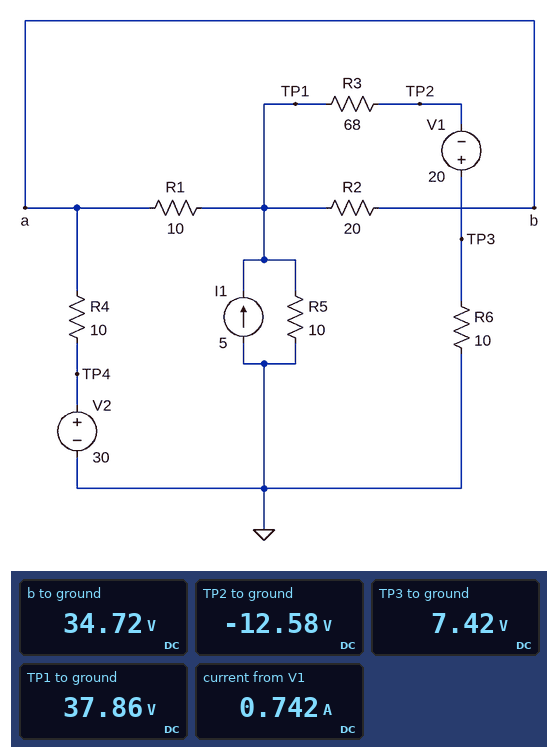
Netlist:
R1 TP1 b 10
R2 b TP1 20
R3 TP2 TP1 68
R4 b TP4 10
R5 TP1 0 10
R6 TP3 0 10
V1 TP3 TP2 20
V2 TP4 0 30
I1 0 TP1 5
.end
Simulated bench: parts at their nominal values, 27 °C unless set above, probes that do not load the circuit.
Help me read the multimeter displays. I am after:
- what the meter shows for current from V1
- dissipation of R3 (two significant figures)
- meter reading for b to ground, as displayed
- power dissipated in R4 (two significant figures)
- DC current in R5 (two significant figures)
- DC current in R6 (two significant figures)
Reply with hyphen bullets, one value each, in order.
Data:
- 0.742 A
- 37 W
- 34.72 V
- 2.2 W
- 3.8 A
- 740 mA
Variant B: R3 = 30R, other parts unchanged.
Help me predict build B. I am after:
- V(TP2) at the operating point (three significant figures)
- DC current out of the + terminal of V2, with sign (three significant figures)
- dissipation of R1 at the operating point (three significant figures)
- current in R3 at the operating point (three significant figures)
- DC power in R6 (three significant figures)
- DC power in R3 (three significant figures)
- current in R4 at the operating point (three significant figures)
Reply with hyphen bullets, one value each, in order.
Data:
- -6.49 V
- -243 mA
- 263 mW
- 1.35 A
- 18.3 W
- 54.8 W
- 243 mA
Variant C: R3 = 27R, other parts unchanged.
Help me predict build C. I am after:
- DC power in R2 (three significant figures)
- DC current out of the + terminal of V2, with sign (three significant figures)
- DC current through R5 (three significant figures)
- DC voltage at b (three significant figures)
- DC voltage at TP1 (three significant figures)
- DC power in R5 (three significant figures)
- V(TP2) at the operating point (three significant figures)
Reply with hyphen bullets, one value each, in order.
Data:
- 96.2 mW
- -208 mA
- 3.35 A
- 32.1 V
- 33.5 V
- 112 W
- -5.55 V
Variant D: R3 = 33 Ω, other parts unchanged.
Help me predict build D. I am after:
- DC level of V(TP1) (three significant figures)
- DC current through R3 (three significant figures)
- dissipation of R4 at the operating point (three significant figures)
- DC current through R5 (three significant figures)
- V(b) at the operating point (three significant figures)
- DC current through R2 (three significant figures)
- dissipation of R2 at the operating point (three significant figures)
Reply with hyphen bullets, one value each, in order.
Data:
- 34.6 V
- 1.27 A
- 751 mW
- 3.46 A
- 32.7 V
- 91.4 mA
- 167 mW
